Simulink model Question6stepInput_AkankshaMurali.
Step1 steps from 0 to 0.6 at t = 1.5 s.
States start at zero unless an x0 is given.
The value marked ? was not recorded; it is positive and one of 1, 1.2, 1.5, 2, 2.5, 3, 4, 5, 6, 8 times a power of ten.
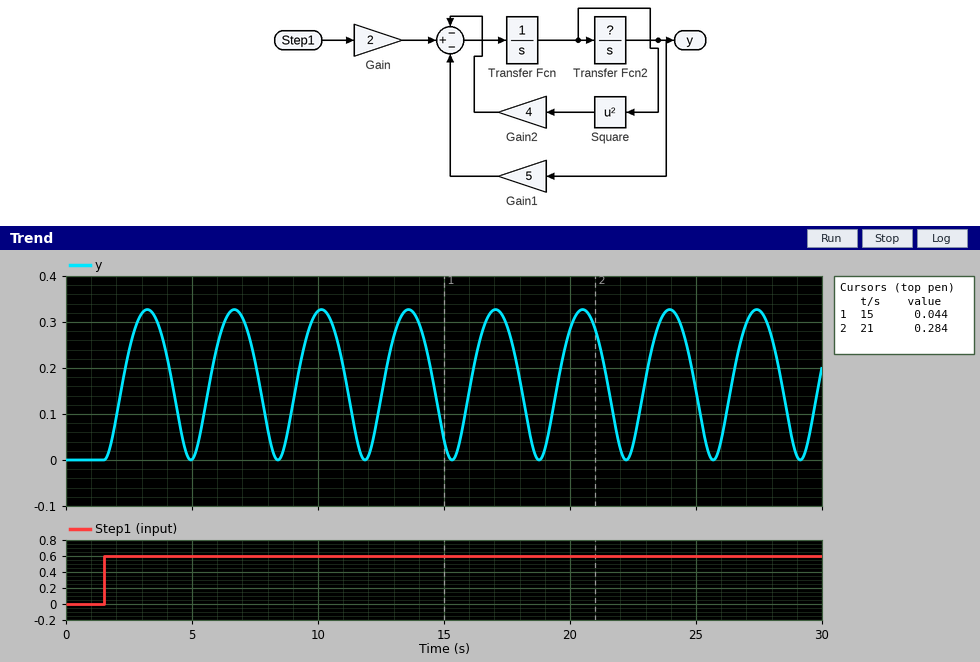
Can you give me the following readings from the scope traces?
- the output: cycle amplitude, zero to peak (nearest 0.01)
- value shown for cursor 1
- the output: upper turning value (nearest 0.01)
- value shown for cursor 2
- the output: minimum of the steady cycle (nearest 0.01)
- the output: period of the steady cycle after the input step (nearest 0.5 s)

0.16
0.044
0.33
0.284
0.00
3.5 s
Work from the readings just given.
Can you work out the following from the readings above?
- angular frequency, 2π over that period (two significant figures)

1.8 rad/s
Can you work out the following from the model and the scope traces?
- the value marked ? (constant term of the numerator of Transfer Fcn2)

0.8
